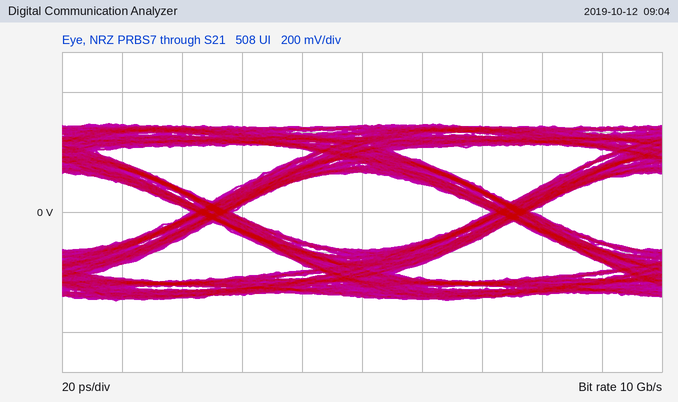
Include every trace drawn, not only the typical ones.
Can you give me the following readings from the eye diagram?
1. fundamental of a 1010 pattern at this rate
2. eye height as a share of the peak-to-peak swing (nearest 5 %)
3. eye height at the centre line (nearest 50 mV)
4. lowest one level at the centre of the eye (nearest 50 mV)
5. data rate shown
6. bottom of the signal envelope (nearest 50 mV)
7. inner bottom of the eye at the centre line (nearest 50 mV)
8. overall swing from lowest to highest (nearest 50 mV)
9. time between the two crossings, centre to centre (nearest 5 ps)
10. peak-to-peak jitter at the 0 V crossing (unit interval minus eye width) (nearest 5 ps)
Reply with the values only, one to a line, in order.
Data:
5 GHz
45 %
400 mV
200 mV
10 Gb/s
-450 mV
-200 mV
900 mV
100 ps
15 ps
